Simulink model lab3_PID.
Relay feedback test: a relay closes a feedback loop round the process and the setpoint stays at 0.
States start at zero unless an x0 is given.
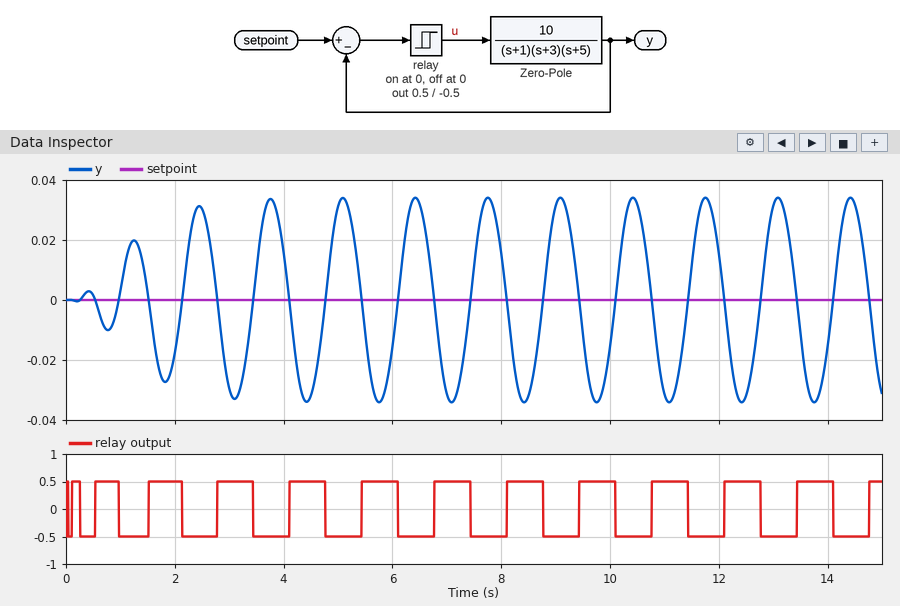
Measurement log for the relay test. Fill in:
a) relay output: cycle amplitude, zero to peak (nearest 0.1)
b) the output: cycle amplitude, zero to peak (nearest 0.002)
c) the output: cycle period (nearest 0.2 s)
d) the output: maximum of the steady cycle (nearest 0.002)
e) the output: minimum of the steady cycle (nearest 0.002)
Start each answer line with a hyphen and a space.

- 0.5
- 0.034
- 1.4 s
- 0.034
- -0.034
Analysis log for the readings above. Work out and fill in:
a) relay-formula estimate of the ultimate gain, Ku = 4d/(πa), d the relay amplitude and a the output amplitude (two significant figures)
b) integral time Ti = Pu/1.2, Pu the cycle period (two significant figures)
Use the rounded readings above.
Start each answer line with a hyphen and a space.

- 19
- 1.2 s
